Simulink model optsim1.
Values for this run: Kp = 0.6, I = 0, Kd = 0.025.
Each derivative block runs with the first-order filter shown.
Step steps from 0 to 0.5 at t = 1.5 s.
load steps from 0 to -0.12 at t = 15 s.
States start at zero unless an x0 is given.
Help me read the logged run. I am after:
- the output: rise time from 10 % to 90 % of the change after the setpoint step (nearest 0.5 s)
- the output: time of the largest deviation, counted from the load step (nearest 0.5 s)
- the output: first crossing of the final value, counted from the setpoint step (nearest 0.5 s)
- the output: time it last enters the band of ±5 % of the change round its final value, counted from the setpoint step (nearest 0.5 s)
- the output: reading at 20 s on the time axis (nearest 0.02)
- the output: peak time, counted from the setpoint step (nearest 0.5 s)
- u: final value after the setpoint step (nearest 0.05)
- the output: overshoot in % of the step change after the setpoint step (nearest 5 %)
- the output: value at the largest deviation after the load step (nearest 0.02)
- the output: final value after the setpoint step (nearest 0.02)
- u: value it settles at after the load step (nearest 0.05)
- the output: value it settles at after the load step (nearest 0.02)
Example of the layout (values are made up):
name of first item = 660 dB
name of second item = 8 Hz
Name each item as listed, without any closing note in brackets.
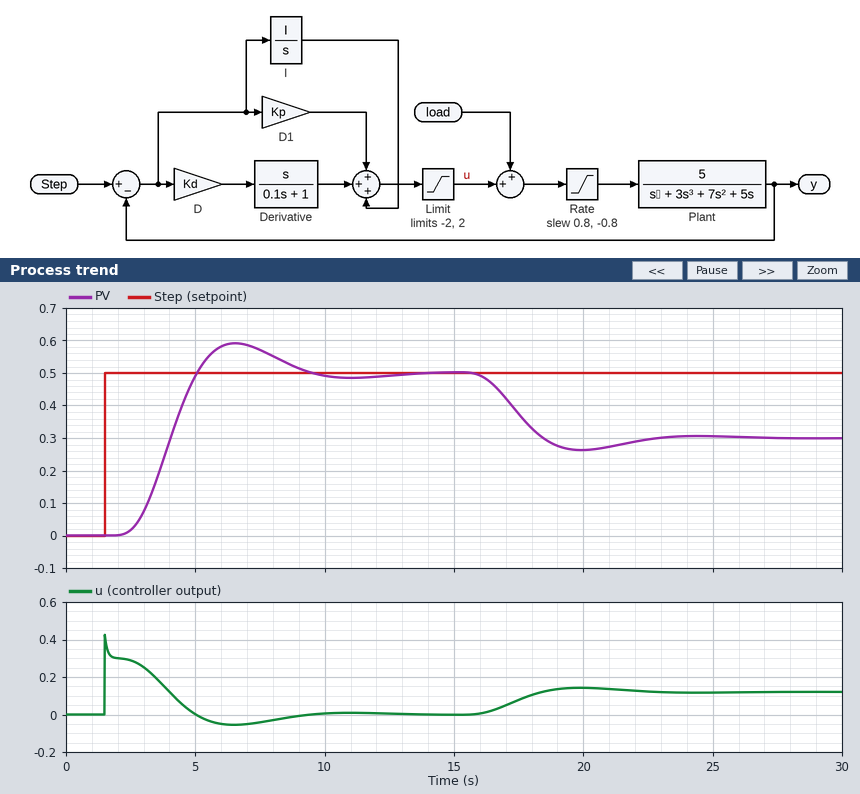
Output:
the output: rise time from 10 % to 90 % of the change after the setpoint step = 2.0 s
the output: time of the largest deviation, counted from the load step = 5.0 s
the output: first crossing of the final value, counted from the setpoint step = 3.5 s
the output: time it last enters the band of ±5 % of the change round its final value, counted from the setpoint step = 7.0 s
the output: reading at 20 s on the time axis = 0.26
the output: peak time, counted from the setpoint step = 5.0 s
u: final value after the setpoint step = 0.00
the output: overshoot in % of the step change after the setpoint step = 20 %
the output: value at the largest deviation after the load step = 0.26
the output: final value after the setpoint step = 0.50
u: value it settles at after the load step = 0.10
the output: value it settles at after the load step = 0.30
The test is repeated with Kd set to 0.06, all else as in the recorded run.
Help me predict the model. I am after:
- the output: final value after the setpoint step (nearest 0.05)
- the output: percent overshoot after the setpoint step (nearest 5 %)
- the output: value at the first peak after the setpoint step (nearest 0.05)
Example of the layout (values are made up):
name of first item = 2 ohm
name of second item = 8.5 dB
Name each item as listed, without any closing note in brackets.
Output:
the output: final value after the setpoint step = 0.50
the output: percent overshoot after the setpoint step = 15 %
the output: value at the first peak after the setpoint step = 0.60
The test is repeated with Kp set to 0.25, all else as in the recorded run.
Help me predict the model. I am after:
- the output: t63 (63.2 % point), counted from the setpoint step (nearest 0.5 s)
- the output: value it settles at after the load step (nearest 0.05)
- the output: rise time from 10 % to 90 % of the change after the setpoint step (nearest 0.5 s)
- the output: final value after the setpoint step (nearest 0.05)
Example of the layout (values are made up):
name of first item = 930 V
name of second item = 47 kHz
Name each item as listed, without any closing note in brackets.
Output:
the output: t63 (63.2 % point), counted from the setpoint step = 4.5 s
the output: value it settles at after the load step = 0.00
the output: rise time from 10 % to 90 % of the change after the setpoint step = 6.0 s
the output: final value after the setpoint step = 0.50
